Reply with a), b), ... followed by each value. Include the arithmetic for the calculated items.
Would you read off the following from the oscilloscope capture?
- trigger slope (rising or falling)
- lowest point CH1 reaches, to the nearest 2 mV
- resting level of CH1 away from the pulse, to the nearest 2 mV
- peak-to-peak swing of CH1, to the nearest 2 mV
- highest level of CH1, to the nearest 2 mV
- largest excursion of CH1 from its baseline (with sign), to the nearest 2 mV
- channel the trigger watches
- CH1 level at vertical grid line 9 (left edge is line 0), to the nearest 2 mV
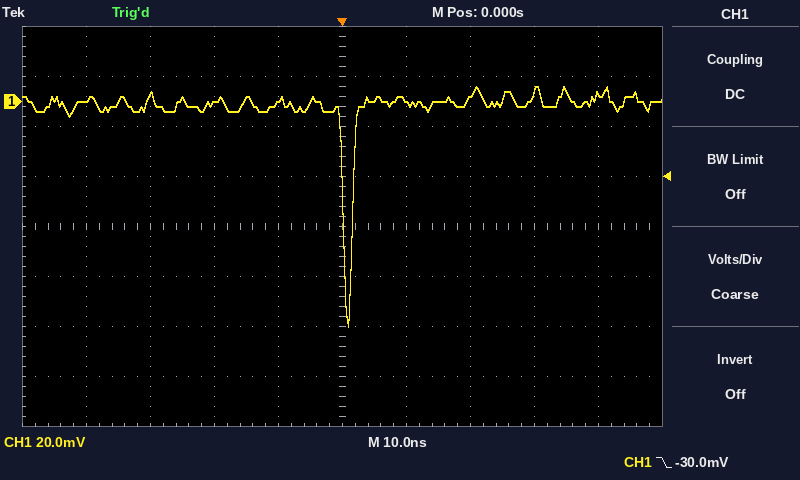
a) falling
b) -90 mV
c) 0 mV
d) 6 mV − (-90 mV) = 96 mV
e) 6 mV
f) -90 mV − (0 mV) = -90 mV
g) CH1
h) 2 mV
